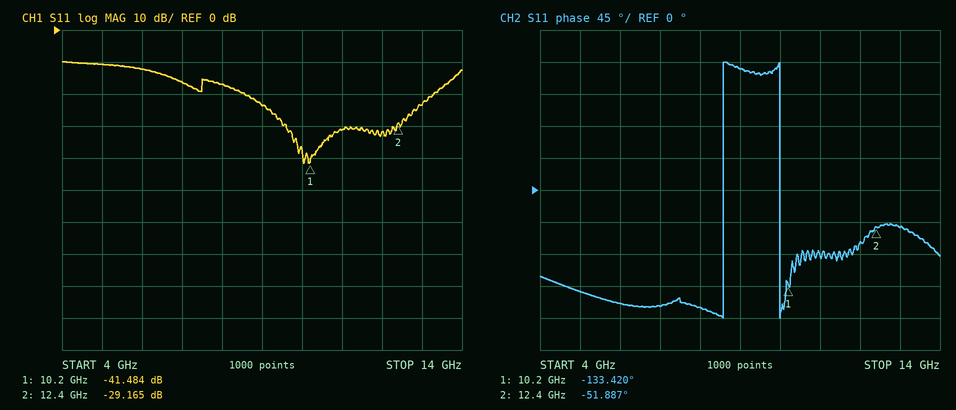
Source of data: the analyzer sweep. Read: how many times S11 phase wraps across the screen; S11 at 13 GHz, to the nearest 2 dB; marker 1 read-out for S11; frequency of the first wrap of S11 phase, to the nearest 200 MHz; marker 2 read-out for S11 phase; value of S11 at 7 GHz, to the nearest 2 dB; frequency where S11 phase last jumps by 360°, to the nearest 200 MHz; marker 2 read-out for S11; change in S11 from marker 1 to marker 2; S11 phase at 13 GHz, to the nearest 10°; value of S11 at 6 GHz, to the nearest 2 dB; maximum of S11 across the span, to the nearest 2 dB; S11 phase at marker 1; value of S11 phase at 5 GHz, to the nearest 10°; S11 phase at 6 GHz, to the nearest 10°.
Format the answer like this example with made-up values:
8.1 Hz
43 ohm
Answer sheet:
2
-24 dB
-41.484 dB
8.6 GHz
-51.887°
-16 dB
10.0 GHz
-29.165 dB
12.319 dB
-50°
-12 dB
-10 dB
-133.420°
-140°
-160°
